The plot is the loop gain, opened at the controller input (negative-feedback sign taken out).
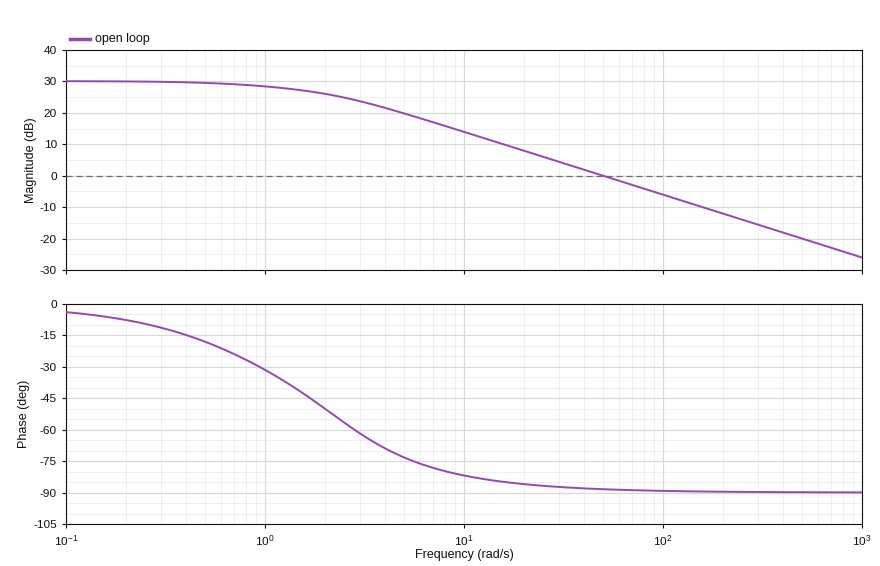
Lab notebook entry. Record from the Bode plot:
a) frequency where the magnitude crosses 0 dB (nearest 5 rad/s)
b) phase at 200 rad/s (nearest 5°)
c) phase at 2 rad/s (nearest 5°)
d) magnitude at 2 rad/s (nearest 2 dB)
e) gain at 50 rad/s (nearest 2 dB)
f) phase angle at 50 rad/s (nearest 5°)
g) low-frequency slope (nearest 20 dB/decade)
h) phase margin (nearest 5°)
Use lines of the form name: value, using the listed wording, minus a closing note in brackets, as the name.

frequency where the magnitude crosses 0 dB: 50 rad/s
phase at 200 rad/s: -90°
phase at 2 rad/s: -50°
magnitude at 2 rad/s: 26 dB
gain at 50 rad/s: 0 dB
phase angle at 50 rad/s: -90°
low-frequency slope: 0 dB/decade
phase margin: 90°
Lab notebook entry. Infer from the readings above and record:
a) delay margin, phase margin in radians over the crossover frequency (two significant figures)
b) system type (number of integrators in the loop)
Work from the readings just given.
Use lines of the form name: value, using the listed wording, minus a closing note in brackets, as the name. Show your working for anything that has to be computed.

delay margin, phase margin in radians over the crossover frequency: 90 × π / 180 / 50 = 0.031 s
system type: 0
